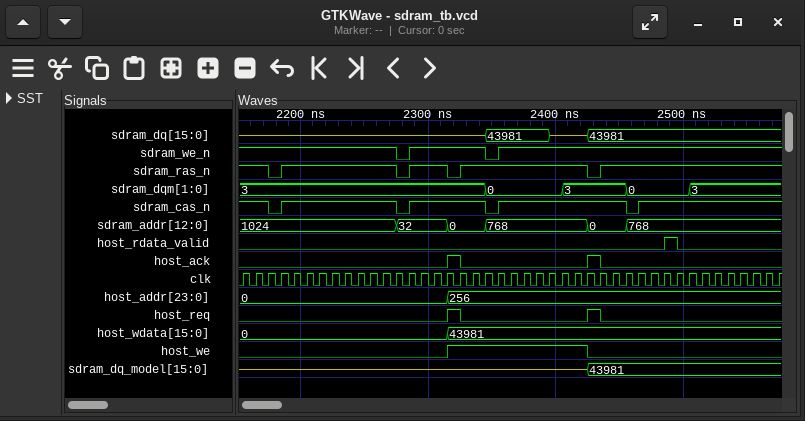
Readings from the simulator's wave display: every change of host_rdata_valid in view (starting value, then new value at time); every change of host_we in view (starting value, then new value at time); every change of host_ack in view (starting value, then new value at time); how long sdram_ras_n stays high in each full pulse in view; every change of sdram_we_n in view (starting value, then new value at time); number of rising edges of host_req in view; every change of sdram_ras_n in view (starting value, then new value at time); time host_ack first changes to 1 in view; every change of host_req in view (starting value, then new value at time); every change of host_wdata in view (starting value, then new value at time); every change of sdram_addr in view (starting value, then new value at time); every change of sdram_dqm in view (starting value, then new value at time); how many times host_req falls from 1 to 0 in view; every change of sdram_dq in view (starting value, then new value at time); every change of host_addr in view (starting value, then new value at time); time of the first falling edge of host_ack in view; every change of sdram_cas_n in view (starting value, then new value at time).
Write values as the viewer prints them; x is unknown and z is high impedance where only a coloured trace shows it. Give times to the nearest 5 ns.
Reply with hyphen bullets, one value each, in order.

- 0, 1 at 2485 ns, 0 at 2495 ns
- 0, 1 at 2315 ns, 0 at 2425 ns
- 0, 1 at 2315 ns, 0 at 2325 ns, 1 at 2425 ns, 0 at 2435 ns
- 90 ns, 30 ns, 100 ns
- 1, 0 at 2275 ns, 1 at 2285 ns, 0 at 2345 ns, 1 at 2355 ns
- 2
- 1, 0 at 2175 ns, 1 at 2185 ns, 0 at 2275 ns, 1 at 2285 ns, 0 at 2315 ns, 1 at 2325 ns, 0 at 2425 ns, 1 at 2435 ns
- 2315 ns
- 0, 1 at 2315 ns, 0 at 2325 ns, 1 at 2425 ns, 0 at 2435 ns
- 0, 43981 at 2315 ns
- 1024, 32 at 2275 ns, 0 at 2315 ns, 768 at 2345 ns, 0 at 2425 ns, 768 at 2455 ns
- 3, 0 at 2345 ns, 3 at 2405 ns, 0 at 2455 ns, 3 at 2505 ns
- 2
- z, 43981 at 2345 ns, z at 2395 ns, 43981 at 2425 ns
- 0, 256 at 2315 ns
- 2325 ns
- 1, 0 at 2175 ns, 1 at 2185 ns, 0 at 2275 ns, 1 at 2285 ns, 0 at 2345 ns, 1 at 2355 ns, 0 at 2455 ns, 1 at 2465 ns
